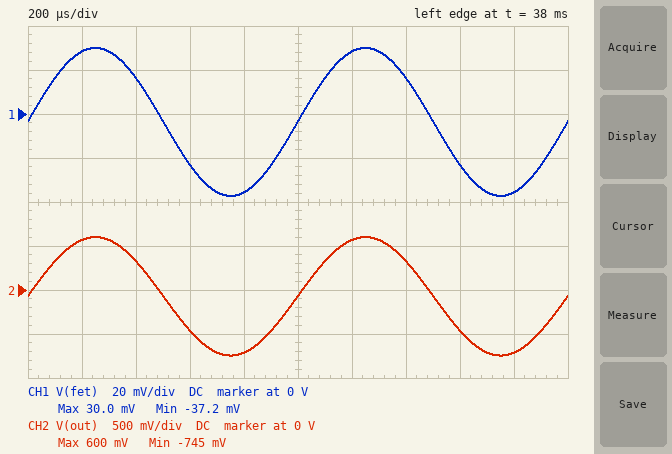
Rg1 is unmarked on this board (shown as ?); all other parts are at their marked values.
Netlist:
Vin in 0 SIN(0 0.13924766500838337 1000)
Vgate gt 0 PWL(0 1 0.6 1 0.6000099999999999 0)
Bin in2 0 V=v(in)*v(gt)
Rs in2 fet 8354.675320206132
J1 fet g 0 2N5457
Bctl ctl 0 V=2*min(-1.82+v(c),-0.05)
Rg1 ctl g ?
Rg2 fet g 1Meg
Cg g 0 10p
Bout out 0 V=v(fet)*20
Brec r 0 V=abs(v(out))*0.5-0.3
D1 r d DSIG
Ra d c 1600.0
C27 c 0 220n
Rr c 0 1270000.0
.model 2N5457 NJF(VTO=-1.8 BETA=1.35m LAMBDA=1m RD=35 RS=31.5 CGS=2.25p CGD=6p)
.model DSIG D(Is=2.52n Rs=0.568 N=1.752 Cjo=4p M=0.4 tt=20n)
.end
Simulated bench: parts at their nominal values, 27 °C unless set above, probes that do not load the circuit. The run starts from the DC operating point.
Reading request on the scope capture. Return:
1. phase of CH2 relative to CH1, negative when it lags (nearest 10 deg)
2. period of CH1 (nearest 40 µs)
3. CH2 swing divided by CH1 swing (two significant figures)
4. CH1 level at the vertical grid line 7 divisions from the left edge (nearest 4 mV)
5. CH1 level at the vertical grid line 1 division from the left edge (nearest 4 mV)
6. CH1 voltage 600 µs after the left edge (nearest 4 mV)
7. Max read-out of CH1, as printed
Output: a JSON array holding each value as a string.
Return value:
["0 deg", "1.00 ms", "20", "16 mV", "28 mV", "-24 mV", "30.0 mV"]
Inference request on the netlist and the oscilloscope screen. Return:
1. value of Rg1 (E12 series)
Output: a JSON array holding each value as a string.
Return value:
["1.2 MΩ"]
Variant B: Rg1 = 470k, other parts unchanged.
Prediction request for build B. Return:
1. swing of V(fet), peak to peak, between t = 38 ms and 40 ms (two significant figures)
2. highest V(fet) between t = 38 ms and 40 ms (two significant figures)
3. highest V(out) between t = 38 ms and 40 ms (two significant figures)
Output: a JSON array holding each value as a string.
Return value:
["220 mV", "110 mV", "2.3 V"]
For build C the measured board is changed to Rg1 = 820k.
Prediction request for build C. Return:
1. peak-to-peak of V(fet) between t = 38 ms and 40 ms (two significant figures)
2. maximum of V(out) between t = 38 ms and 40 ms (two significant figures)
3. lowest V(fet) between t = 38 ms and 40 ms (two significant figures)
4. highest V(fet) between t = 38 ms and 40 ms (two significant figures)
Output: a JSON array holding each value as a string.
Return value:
["150 mV", "1.4 V", "-81 mV", "71 mV"]
